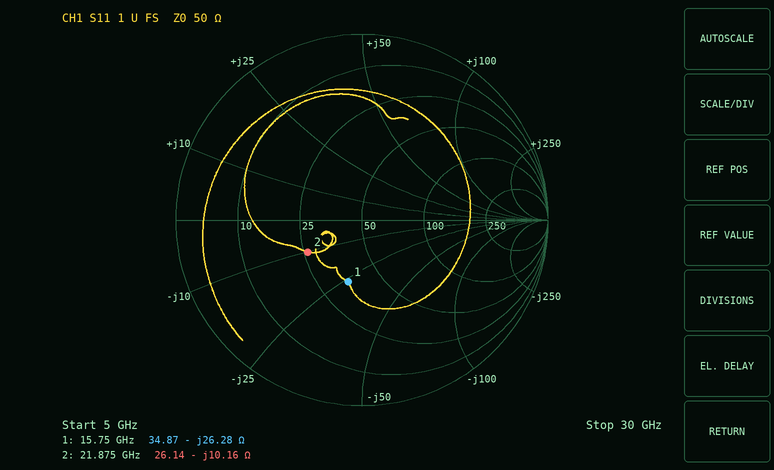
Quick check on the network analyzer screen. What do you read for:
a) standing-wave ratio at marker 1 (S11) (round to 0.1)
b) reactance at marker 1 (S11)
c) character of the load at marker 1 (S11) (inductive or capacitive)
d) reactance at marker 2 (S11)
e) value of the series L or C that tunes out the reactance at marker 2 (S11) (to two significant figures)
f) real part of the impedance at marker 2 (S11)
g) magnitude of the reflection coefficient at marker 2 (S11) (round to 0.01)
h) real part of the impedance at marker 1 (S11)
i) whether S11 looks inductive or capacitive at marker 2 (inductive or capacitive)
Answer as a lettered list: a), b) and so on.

a) 2.0
b) -26.28 Ω
c) capacitive
d) -10.16 Ω
e) 74 pH
f) 26.14 Ω
g) 0.34
h) 34.87 Ω
i) capacitive
